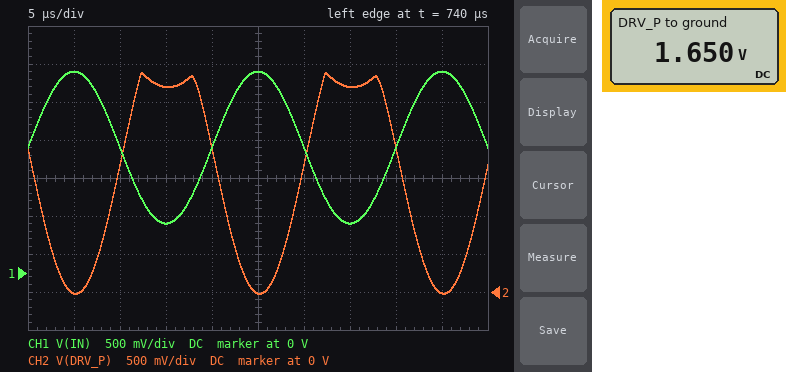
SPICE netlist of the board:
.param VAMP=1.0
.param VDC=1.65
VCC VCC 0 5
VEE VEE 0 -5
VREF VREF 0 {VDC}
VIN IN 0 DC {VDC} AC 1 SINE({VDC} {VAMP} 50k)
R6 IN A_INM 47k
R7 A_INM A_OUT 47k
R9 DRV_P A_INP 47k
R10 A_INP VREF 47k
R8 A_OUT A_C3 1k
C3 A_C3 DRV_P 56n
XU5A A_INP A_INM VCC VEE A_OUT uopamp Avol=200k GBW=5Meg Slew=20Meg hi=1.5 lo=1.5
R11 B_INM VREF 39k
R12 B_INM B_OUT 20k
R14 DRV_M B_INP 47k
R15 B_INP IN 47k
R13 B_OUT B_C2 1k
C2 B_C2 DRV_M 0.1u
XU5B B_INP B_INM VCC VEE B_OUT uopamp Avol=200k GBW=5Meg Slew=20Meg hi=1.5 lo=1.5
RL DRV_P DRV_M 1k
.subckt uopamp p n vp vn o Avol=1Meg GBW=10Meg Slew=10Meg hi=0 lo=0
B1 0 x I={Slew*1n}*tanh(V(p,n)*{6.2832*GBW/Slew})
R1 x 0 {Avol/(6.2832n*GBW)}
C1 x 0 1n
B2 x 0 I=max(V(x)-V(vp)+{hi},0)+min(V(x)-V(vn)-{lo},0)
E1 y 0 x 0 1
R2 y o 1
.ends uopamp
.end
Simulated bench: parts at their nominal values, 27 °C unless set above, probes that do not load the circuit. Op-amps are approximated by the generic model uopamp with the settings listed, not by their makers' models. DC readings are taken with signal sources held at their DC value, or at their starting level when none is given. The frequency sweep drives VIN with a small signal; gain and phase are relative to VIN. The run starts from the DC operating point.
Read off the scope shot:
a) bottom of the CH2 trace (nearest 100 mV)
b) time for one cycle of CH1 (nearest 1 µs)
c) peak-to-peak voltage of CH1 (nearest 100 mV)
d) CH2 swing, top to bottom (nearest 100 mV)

0 V
20 µs
2.0 V
2.9 V
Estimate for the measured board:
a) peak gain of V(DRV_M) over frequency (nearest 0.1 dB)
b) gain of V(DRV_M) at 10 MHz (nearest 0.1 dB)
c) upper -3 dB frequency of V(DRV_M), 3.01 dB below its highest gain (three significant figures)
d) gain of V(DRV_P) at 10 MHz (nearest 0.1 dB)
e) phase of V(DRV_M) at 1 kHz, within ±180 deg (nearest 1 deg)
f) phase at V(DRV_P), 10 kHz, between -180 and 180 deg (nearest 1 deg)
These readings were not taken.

-1.5 dB
-21.4 dB
421 kHz
-21.9 dB
-36 deg
-158 deg
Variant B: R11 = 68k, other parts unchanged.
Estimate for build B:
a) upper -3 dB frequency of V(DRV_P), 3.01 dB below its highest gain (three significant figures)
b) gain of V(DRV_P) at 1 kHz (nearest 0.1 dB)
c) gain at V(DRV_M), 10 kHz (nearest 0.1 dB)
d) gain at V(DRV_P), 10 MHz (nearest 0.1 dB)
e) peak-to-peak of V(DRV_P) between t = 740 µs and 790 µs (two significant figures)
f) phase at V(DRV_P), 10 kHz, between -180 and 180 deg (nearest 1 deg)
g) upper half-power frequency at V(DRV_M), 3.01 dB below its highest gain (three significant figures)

465 kHz
-3.1 dB
-1.3 dB
-21.7 dB
3.0 V
-163 deg
527 kHz
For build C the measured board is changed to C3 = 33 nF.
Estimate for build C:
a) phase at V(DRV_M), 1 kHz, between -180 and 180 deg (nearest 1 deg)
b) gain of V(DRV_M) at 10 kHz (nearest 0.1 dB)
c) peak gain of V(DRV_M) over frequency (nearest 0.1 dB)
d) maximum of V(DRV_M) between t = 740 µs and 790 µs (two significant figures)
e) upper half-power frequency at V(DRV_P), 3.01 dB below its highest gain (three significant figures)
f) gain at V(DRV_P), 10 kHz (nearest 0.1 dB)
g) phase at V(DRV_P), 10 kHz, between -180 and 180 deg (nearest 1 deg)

-13 deg
0.4 dB
4.3 dB
2.3 V
344 kHz
5.1 dB
-132 deg
